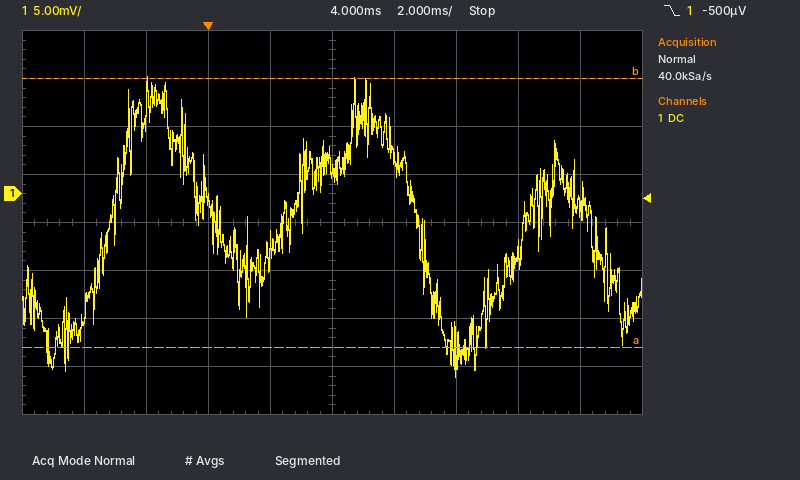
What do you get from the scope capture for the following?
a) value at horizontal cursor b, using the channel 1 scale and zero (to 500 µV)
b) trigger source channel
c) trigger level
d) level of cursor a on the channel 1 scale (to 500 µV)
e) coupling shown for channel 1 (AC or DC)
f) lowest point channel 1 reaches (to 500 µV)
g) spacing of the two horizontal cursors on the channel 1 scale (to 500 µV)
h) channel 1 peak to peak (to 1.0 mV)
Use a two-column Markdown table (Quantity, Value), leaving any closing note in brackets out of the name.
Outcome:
| Quantity | Value |
|---|---|
| value at horizontal cursor b, using the channel 1 scale and zero | 12.0 mV |
| trigger source channel | channel 1 |
| trigger level | -500 µV |
| level of cursor a on the channel 1 scale | -16.0 mV |
| coupling shown for channel 1 | DC |
| lowest point channel 1 reaches | -19.0 mV |
| spacing of the two horizontal cursors on the channel 1 scale | 28.0 mV |
| channel 1 peak to peak | 31.0 mV |
